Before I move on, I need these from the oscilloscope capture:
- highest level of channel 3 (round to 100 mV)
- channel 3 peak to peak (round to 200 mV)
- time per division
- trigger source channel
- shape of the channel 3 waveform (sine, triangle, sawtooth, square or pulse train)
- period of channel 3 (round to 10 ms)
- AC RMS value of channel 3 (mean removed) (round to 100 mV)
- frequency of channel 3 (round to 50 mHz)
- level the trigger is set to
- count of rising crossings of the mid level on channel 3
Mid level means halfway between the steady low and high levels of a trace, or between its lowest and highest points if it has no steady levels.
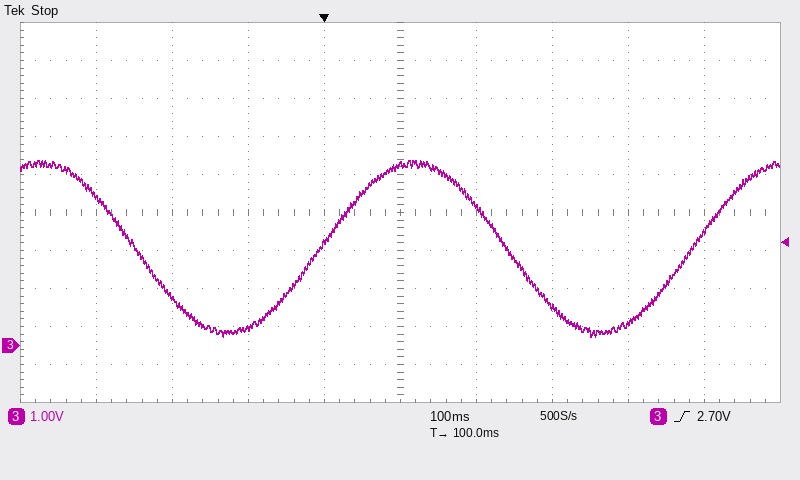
4.9 V
4.6 V
100 ms
channel 3
sine
490 ms
1.6 V
2.05 Hz
2.70 V
2
